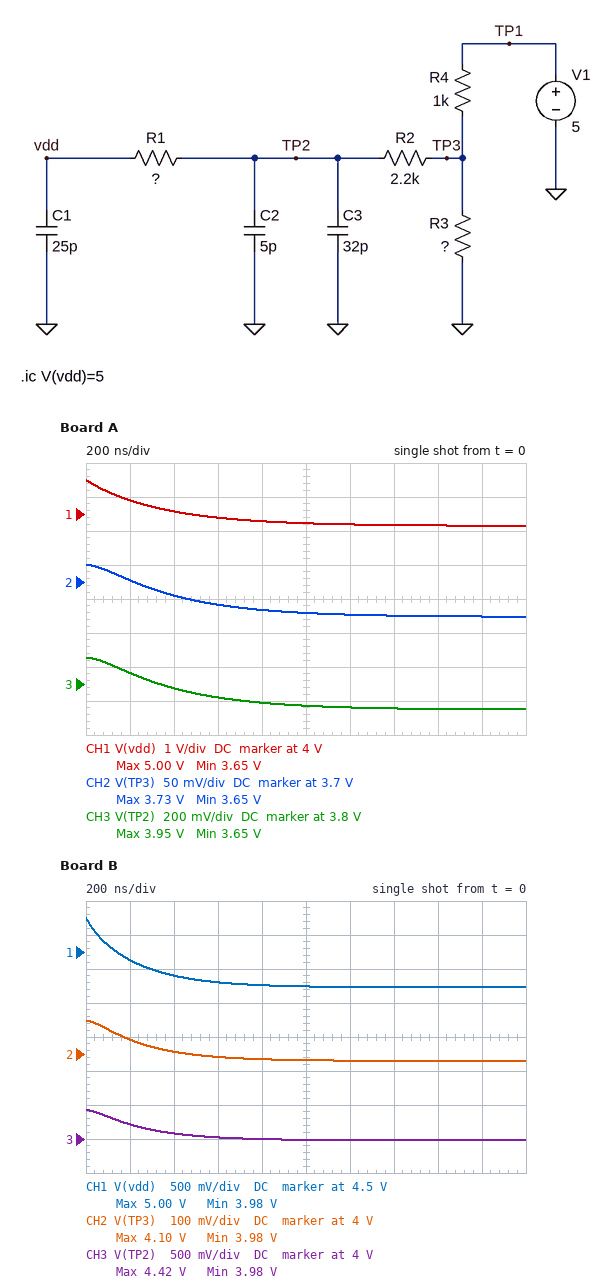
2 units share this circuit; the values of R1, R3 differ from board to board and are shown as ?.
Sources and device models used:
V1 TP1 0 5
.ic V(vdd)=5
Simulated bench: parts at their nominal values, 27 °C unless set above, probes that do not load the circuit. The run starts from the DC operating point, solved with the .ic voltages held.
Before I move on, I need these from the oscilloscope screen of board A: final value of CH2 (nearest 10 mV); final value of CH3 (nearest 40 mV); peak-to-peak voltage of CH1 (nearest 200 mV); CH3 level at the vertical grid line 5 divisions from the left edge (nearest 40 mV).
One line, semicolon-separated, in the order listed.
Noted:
3.65 V; 3.64 V; 1.4 V; 3.68 V
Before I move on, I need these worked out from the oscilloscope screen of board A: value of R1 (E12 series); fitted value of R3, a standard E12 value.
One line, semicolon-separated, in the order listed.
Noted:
10 kΩ; 2.7 kΩ
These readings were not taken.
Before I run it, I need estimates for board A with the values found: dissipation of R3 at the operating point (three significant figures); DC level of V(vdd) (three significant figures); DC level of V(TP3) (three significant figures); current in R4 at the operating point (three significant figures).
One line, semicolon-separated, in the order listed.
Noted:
4.93 mW; 3.65 V; 3.65 V; 1.35 mA
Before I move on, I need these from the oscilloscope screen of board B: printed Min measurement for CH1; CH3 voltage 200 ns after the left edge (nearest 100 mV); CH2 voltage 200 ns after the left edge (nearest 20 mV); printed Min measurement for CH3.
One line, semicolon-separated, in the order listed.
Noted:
3.98 V; 4.2 V; 4.04 V; 3.98 V
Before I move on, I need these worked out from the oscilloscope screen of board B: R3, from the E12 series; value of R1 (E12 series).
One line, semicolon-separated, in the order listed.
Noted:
3.9 kΩ; 3.9 kΩ
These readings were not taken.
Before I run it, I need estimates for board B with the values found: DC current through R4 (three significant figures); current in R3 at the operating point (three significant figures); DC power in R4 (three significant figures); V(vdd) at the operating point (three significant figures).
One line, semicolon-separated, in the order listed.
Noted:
1.02 mA; 1.02 mA; 1.04 mW; 3.98 V
